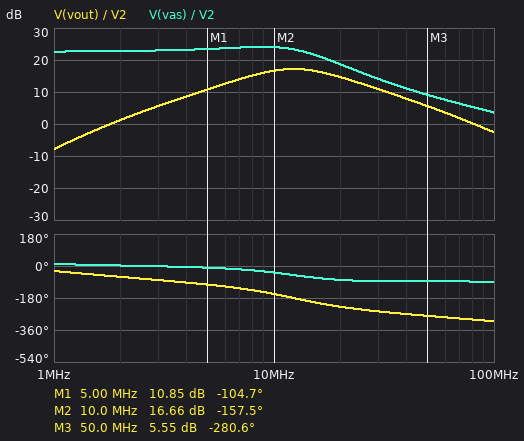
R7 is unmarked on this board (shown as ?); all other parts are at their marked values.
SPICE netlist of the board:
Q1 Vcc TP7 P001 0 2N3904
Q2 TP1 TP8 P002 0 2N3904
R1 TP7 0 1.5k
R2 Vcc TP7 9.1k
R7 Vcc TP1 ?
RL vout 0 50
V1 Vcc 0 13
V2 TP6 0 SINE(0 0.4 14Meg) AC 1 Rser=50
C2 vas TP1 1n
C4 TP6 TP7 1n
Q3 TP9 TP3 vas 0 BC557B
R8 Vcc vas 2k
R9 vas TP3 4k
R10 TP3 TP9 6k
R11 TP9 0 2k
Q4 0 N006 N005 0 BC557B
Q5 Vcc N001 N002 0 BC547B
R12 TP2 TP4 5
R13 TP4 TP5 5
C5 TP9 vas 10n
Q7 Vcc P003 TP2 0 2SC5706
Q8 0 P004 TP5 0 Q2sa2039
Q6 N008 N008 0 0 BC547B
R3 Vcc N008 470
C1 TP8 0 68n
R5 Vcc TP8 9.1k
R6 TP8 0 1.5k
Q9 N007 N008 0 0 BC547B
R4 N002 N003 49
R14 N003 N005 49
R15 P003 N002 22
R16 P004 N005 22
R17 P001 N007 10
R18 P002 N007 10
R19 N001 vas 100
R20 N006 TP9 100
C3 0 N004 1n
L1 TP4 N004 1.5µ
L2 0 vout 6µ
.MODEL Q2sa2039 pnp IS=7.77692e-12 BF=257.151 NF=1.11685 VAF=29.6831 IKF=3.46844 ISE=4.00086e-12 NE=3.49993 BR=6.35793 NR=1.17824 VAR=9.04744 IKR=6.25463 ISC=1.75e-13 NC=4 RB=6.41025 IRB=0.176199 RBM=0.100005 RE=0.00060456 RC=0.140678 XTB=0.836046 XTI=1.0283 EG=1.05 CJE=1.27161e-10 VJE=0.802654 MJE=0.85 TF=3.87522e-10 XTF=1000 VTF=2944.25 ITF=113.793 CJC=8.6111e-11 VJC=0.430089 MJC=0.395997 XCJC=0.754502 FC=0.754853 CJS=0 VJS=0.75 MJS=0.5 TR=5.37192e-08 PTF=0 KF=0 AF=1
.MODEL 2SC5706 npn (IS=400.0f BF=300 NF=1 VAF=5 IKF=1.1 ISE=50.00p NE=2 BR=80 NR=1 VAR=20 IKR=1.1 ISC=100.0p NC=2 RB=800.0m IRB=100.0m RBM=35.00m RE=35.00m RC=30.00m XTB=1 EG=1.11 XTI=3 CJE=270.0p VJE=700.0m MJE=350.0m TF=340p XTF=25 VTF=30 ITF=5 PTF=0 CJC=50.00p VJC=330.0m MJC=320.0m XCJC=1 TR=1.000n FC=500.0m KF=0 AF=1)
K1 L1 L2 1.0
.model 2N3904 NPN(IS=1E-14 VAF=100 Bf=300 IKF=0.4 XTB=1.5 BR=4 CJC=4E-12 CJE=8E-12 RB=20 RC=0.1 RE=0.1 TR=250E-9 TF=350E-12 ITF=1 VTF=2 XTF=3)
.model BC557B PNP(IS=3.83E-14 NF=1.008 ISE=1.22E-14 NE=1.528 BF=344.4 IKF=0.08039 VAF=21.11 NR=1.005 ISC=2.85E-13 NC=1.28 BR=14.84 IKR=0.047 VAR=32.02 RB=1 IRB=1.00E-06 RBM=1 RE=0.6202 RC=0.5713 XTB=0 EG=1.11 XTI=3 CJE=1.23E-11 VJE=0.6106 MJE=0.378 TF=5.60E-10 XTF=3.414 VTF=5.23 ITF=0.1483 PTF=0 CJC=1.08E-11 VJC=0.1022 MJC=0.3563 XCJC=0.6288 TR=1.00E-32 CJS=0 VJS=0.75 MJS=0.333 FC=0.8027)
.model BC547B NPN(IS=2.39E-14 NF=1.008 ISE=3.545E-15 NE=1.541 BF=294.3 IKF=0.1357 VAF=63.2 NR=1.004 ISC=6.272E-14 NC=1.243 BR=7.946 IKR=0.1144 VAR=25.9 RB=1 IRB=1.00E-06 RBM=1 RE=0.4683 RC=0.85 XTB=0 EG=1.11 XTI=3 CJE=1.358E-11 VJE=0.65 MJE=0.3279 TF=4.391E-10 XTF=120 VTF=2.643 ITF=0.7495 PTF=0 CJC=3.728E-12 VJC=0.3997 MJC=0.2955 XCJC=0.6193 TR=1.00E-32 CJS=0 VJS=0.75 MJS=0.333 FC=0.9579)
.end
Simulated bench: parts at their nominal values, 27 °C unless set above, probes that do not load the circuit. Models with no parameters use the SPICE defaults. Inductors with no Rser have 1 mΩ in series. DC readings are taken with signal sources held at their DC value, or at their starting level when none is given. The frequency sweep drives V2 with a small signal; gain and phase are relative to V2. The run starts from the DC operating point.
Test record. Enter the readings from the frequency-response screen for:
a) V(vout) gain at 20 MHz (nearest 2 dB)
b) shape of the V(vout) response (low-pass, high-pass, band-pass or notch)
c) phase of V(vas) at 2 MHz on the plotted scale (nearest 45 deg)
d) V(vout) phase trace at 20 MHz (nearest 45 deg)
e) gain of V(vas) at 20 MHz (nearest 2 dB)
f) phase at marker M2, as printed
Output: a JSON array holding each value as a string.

["14 dB", "band-pass", "0 deg", "-225 deg", "18 dB", "-157.5 deg"]
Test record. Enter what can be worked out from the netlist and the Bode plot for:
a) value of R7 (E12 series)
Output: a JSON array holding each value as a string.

["560 Ω"]
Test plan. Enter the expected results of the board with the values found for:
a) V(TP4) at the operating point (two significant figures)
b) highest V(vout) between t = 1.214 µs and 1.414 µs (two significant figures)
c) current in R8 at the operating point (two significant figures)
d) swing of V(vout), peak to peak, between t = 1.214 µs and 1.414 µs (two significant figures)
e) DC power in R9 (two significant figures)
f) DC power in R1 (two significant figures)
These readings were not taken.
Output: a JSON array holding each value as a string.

["6.5 V", "7.5 V", "2.8 mA", "16 V", "110 µW", "2.1 mW"]
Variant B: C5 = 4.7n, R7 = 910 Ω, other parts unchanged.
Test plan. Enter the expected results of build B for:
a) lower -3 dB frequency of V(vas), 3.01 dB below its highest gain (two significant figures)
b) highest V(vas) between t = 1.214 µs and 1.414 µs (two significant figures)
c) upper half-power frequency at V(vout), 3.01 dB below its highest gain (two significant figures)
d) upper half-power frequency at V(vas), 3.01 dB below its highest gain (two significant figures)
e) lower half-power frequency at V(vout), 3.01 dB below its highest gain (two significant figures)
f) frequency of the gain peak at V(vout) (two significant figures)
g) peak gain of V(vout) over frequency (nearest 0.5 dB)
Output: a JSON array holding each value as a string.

["220 kHz", "8.9 V", "18 MHz", "13 MHz", "6.0 MHz", "10 MHz", "18.0 dB"]
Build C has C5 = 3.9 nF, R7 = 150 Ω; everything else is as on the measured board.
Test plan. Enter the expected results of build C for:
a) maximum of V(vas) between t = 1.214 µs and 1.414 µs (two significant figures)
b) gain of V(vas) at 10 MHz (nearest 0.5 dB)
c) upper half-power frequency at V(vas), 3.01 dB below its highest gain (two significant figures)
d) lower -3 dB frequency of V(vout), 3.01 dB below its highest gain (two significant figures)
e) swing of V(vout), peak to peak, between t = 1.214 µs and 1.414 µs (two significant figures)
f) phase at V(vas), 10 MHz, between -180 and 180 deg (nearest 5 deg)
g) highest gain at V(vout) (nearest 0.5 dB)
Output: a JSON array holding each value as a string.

["9.5 V", "14.5 dB", "28 MHz", "9.2 MHz", "5.2 V", "-15 deg", "9.5 dB"]
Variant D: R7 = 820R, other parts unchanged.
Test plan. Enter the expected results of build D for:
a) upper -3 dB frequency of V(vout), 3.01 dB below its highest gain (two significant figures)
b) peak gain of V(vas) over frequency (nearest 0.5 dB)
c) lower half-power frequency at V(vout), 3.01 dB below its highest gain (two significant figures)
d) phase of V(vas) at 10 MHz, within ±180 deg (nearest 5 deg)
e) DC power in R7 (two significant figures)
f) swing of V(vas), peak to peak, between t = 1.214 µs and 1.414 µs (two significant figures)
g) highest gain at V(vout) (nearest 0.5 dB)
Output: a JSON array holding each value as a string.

["19 MHz", "26.0 dB", "6.4 MHz", "-50 deg", "130 mW", "5.6 V", "18.5 dB"]
